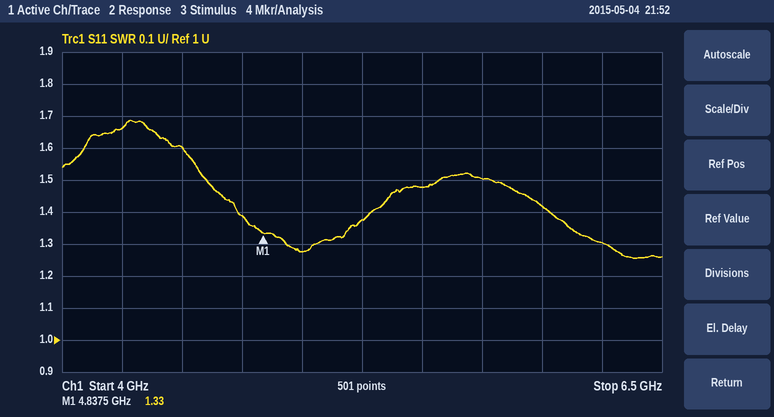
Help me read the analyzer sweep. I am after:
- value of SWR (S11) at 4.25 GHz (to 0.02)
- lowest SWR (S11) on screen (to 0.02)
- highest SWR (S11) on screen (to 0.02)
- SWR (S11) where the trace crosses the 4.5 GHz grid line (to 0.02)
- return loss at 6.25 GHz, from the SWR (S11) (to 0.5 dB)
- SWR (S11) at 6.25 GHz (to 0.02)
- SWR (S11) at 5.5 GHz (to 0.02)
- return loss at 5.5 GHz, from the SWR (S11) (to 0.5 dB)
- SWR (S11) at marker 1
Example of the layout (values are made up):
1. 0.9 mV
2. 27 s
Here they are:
1. 1.66
2. 1.26
3. 1.68
4. 1.60
5. 17.5 dB
6. 1.30
7. 1.48
8. 14.5 dB
9. 1.33
